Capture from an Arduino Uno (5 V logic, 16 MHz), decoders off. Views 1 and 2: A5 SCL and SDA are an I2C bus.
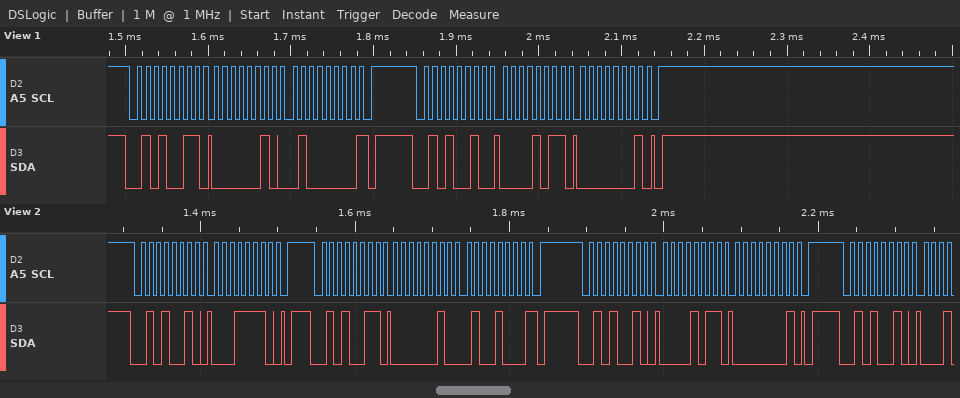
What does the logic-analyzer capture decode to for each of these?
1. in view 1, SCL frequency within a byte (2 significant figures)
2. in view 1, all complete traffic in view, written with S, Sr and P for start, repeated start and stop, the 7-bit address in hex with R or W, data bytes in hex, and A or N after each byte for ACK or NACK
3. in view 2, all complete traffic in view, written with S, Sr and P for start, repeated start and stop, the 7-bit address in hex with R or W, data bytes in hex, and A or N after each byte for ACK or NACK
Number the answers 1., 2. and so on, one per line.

1. 100 kHz
2. S 29R A 02 A 40 N P S 29W A 0B A 01 A P
3. S 29W A 1E A P S 29R A 02 A 48 N P S 29W A 0B A 01 A P S 29W A
